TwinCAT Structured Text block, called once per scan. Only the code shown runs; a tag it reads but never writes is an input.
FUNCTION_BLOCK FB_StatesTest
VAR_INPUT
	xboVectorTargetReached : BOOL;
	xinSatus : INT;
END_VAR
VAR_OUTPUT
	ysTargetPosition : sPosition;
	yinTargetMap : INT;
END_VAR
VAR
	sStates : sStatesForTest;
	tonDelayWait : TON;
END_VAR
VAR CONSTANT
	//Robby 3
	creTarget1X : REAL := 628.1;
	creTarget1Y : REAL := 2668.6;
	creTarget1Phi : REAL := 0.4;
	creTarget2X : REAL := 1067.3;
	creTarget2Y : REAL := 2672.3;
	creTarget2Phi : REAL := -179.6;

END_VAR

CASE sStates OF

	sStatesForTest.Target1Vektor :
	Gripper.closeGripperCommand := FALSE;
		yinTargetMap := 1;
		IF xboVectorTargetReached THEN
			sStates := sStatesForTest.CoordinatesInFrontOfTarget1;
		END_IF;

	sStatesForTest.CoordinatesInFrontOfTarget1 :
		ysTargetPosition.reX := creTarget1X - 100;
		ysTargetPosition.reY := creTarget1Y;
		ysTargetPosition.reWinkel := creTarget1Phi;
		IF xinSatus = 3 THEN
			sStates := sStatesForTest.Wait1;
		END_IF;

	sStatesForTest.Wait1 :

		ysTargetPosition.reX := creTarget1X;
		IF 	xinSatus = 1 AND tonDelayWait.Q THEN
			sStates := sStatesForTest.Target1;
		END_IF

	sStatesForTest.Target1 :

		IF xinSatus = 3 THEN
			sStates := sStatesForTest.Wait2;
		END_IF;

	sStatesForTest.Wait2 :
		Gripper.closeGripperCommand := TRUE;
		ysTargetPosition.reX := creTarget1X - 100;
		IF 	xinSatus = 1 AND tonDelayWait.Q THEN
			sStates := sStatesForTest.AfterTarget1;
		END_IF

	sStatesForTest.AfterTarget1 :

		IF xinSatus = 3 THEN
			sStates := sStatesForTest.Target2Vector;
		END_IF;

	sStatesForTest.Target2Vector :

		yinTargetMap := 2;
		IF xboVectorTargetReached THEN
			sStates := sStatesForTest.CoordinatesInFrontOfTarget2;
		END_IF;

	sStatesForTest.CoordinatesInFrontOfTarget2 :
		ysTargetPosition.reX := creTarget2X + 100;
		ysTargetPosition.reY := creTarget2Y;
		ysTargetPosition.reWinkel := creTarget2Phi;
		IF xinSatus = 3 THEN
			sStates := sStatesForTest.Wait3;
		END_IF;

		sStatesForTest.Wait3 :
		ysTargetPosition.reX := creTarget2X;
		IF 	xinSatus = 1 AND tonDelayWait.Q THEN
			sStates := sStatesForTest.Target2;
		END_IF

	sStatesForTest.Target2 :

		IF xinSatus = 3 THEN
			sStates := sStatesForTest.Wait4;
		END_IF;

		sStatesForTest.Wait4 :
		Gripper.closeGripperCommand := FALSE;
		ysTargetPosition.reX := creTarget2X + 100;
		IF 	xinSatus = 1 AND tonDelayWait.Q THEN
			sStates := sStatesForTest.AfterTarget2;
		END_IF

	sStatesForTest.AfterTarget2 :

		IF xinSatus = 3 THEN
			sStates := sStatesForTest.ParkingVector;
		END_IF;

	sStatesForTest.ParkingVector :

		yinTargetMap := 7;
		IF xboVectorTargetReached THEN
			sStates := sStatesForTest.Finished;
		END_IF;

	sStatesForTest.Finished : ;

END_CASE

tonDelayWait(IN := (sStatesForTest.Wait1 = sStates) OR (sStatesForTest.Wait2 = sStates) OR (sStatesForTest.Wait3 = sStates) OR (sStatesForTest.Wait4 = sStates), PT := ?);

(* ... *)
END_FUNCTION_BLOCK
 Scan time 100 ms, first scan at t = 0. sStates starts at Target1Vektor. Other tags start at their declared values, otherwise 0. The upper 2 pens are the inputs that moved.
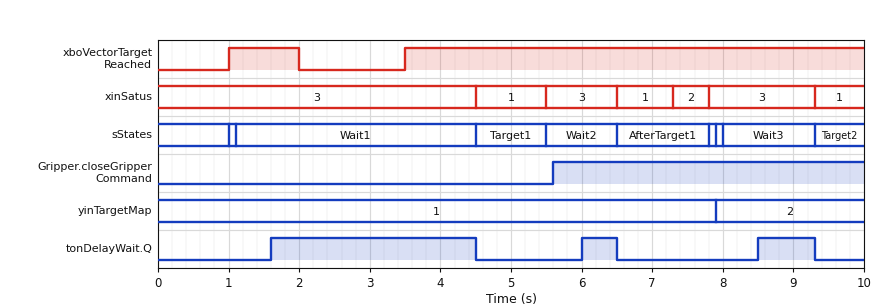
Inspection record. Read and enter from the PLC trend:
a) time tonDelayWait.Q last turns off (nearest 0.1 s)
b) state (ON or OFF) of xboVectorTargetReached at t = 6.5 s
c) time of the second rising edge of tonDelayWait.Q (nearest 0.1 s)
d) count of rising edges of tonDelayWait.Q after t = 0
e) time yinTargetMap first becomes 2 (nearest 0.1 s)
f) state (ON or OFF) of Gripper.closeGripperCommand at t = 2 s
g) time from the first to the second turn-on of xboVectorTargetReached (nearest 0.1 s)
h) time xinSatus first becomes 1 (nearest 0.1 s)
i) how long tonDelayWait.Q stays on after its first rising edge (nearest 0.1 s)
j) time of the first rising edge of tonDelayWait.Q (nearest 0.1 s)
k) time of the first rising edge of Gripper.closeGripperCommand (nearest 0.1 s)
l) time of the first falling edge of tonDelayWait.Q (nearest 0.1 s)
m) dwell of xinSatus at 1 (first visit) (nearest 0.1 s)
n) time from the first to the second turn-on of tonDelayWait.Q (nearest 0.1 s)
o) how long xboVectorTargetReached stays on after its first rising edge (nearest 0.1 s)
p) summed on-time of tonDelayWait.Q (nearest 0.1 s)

9.3 s
ON
6.0 s
3
7.9 s
OFF
2.5 s
4.5 s
2.9 s
1.6 s
5.6 s
4.5 s
1.0 s
4.4 s
1.0 s
4.2 s
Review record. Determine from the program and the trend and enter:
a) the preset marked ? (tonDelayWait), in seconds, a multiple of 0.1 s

0.5 s
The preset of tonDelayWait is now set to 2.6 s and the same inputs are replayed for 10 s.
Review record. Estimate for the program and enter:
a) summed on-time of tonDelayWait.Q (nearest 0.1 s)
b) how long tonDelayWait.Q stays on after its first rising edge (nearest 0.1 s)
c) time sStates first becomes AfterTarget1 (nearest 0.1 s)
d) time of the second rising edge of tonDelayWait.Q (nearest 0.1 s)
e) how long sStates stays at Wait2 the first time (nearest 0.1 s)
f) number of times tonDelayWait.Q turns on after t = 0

2.0 s
0.8 s
9.3 s
8.1 s
3.8 s
2
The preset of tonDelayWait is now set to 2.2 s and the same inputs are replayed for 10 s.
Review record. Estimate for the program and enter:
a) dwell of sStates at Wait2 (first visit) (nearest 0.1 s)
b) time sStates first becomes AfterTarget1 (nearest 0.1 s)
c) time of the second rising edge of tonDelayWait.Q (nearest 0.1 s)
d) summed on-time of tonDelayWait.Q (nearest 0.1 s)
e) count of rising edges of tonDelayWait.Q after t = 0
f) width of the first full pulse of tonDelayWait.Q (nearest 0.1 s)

3.8 s
9.3 s
7.7 s
2.8 s
2
1.2 s
